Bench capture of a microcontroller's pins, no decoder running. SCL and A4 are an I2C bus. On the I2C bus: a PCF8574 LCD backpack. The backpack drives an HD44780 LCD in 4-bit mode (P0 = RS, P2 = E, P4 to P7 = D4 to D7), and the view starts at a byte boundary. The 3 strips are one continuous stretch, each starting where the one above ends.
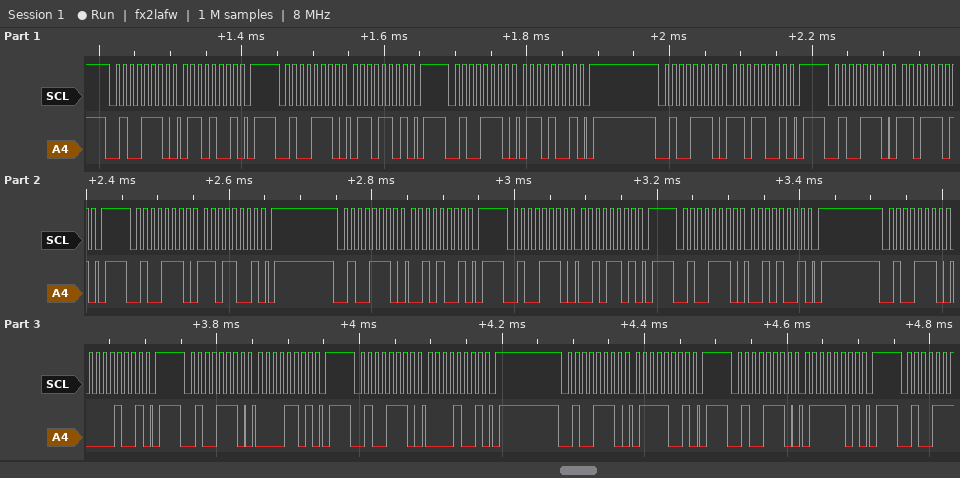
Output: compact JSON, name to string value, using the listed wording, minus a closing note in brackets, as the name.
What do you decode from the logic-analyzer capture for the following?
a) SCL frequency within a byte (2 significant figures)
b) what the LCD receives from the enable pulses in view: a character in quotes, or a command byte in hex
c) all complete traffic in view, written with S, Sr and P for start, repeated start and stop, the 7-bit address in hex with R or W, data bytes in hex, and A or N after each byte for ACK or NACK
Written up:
{"SCL frequency within a byte": "100 kHz", "what the LCD receives from the enable pulses in view: a character in quotes, or a command byte in hex": "'m' ' '", "all complete traffic in view, written with S, Sr and P for start, repeated start and stop, the 7-bit address in hex with R or W, data bytes in hex, and A or N after each byte for ACK or NACK": "S 27W A 69 A P S 27W A 6D A P S 27W A 69 A P S 27W A D9 A P S 27W A DD A P S 27W A D9 A P S 27W A 29 A P S 27W A 2D A P S 27W A 29 A P S 27W A 09 A P S 27W A 0D A P S 27W A 09 A P S 27W A 79 A P S 27W A 7D A P"}
